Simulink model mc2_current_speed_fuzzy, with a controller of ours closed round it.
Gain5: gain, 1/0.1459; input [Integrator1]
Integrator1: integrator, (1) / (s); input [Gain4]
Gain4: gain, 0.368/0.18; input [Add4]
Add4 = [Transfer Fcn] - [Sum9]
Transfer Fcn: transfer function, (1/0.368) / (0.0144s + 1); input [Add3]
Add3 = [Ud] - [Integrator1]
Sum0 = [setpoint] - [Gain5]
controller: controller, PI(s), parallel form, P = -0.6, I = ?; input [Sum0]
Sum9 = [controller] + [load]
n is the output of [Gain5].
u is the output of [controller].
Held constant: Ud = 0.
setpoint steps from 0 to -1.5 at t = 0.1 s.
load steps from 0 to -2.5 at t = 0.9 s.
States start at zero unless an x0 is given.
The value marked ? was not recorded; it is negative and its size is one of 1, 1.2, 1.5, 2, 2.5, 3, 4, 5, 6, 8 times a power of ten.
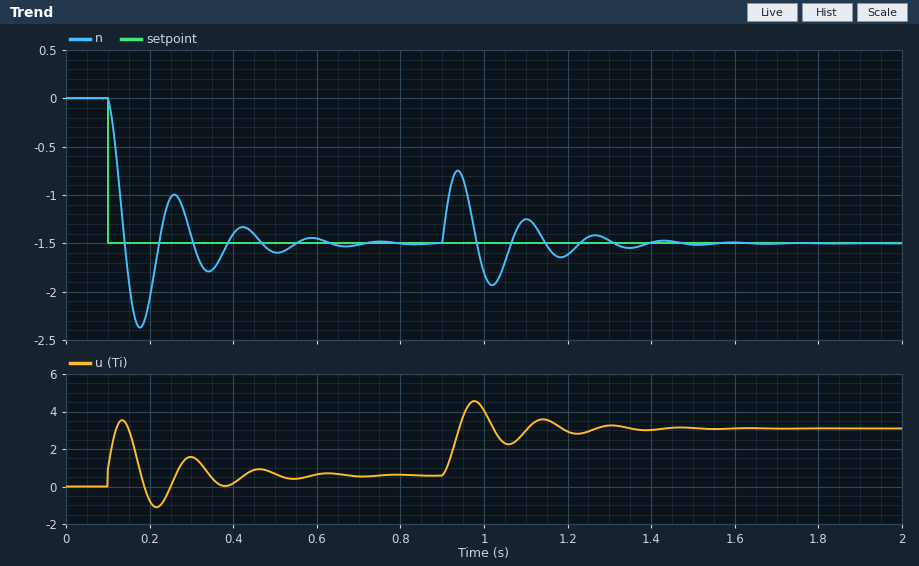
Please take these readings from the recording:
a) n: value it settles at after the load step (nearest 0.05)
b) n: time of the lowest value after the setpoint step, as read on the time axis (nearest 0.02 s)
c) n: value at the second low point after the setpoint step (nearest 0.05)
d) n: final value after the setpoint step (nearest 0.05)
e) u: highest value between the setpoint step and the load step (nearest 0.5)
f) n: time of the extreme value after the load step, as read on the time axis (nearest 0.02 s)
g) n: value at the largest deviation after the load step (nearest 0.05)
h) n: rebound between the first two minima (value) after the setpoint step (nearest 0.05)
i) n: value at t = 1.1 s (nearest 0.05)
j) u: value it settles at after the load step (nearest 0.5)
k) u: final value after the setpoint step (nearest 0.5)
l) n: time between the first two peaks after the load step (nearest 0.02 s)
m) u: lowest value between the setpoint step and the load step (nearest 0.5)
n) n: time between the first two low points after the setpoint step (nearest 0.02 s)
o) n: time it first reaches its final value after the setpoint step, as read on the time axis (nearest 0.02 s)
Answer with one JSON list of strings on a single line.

["-1.50", "0.18 s", "-1.80", "-1.50", "3.5", "0.94 s", "-0.75", "-1.00", "-1.25", "3.0", "0.5", "0.16 s", "-1.0", "0.16 s", "0.14 s"]
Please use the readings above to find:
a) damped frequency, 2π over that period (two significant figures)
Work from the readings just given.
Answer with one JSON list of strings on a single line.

["39 rad/s"]
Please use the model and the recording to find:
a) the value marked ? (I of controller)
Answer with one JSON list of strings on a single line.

["-100"]
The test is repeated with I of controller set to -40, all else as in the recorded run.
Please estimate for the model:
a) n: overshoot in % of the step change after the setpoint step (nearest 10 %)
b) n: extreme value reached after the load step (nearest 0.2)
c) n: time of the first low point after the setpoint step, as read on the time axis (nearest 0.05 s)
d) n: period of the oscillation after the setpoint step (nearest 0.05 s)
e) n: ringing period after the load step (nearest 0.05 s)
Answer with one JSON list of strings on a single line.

["40 %", "-0.4", "0.20 s", "0.25 s", "0.25 s"]
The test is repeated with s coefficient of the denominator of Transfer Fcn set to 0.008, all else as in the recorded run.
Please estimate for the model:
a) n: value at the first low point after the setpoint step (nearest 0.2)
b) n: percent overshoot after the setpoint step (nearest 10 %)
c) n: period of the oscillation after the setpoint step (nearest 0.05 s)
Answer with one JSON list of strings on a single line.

["-2.4", "60 %", "0.15 s"]
